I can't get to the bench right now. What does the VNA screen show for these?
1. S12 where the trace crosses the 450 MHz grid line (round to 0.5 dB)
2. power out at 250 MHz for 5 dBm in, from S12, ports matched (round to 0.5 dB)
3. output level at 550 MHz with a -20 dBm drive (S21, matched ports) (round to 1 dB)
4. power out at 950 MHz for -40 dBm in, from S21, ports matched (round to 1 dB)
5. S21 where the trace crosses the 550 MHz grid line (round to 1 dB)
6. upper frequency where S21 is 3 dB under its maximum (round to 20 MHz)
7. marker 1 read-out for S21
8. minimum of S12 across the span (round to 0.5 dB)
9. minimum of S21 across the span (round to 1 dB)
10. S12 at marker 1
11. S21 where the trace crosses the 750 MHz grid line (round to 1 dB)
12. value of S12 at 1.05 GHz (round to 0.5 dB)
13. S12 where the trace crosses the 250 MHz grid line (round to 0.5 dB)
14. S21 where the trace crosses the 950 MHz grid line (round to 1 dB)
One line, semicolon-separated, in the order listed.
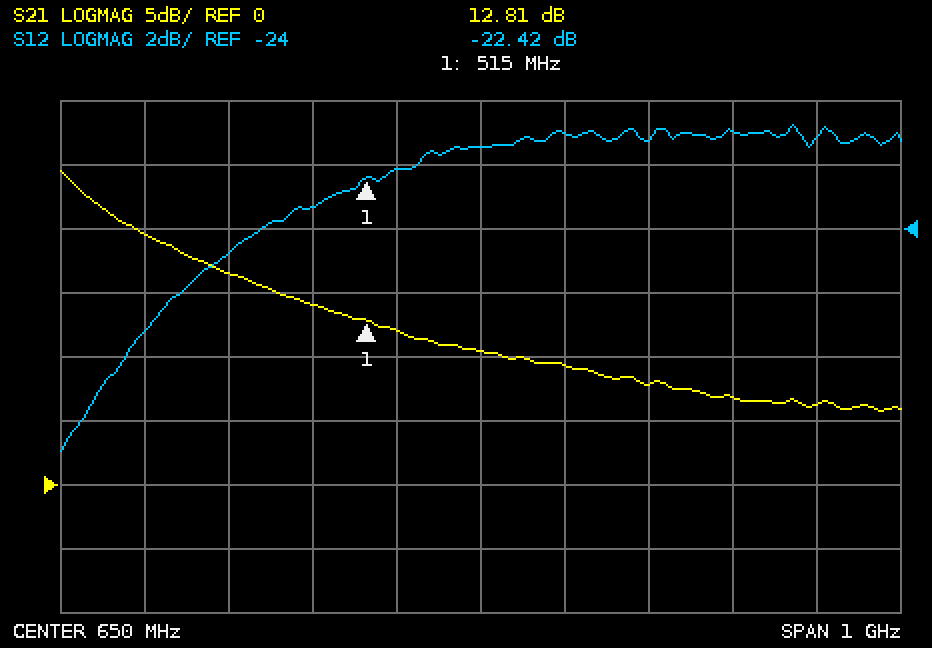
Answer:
-23.5 dB; -22.0 dBm; -8 dBm; -33 dBm; 12 dB; 200 MHz; 12.81 dB; -31.0 dB; 6 dB; -22.42 dB; 9 dB; -21.0 dB; -27.0 dB; 7 dB
